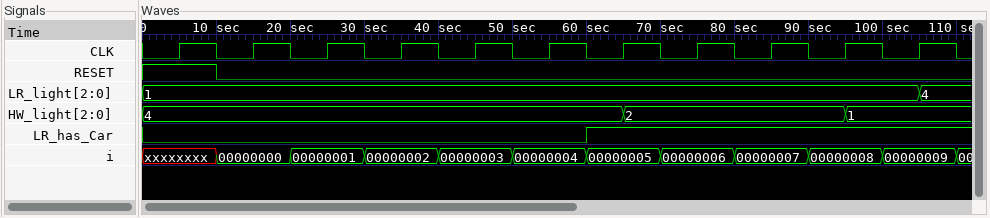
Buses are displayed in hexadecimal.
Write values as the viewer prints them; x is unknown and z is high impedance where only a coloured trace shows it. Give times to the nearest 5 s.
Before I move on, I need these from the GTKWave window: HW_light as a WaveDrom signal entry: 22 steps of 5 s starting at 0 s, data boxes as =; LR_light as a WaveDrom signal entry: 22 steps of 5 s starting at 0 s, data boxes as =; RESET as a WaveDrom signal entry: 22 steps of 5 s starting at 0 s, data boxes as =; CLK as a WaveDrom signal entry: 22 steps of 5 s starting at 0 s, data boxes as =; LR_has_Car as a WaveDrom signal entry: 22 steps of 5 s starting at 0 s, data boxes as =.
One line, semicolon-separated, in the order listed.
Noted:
{name: 'HW_light', wave: '=............=.....=..', data: '4 2 1'}; {name: 'LR_light', wave: '=....................=', data: '1 4'}; {name: 'RESET', wave: '1.0...................'}; {name: 'CLK', wave: '0101010101010101010101'}; {name: 'LR_has_Car', wave: '0...........1.........'}
